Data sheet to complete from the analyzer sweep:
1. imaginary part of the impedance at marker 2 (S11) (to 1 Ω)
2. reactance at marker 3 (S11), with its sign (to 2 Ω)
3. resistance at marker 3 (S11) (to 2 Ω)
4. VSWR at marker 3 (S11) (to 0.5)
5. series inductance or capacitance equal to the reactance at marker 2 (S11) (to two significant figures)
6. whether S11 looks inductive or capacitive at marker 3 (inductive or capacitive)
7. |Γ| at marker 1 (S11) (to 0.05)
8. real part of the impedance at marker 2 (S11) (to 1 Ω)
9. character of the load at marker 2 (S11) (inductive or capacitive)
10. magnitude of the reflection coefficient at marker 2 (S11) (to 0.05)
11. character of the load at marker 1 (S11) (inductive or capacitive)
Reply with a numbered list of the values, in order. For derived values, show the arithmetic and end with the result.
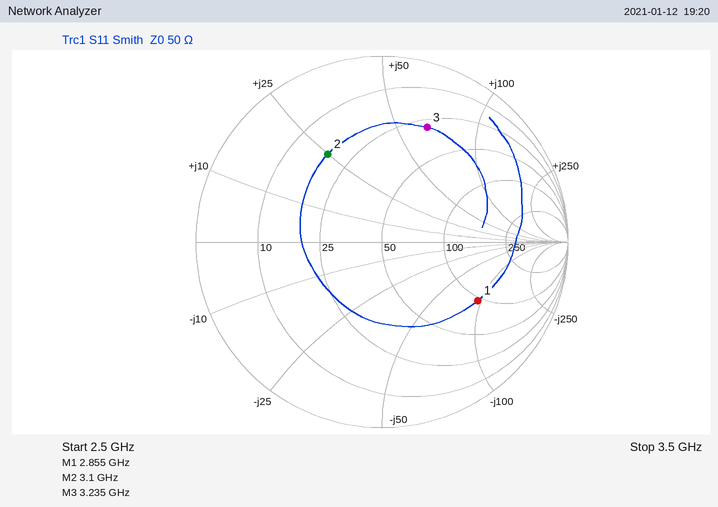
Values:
1. +25 Ω
2. +64 Ω
3. 30 Ω
4. 5.0
5. L = 25 Ω/(2π × 3.1 GHz) ≈ 1.3 nH
6. inductive
7. 0.60
8. 18 Ω
9. inductive
10. 0.55
11. capacitive
